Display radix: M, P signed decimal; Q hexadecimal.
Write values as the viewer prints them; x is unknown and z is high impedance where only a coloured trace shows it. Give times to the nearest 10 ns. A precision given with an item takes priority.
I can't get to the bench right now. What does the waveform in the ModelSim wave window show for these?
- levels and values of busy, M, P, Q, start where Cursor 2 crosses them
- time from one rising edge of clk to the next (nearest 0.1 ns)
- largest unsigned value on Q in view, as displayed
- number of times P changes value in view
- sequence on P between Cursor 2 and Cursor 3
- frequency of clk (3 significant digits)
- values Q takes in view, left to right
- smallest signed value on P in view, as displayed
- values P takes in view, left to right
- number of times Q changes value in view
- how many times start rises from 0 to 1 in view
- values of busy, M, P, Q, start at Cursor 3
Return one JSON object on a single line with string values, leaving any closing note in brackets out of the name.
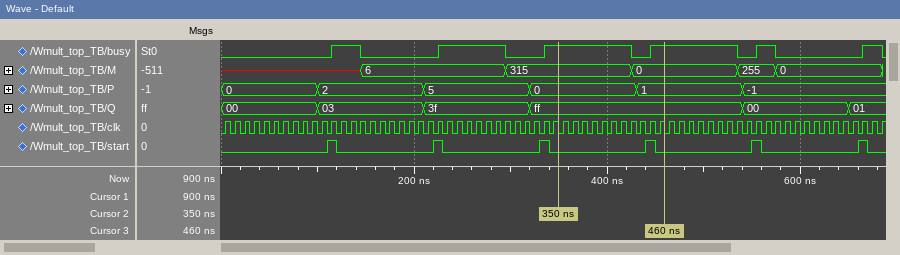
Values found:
{"levels and values of busy, M, P, Q, start where Cursor 2 crosses them": "busy=1, M=315, P=0, Q=ff, start=0", "time from one rising edge of clk to the next": "10 ns", "largest unsigned value on Q in view, as displayed": "ff", "number of times P changes value in view": "5", "sequence on P between Cursor 2 and Cursor 3": "0, 1", "frequency of clk": "100 MHz", "values Q takes in view, left to right": "00, 03, 3f, ff, 00, 01", "smallest signed value on P in view, as displayed": "-1", "values P takes in view, left to right": "0, 2, 5, 0, 1, -1", "number of times Q changes value in view": "5", "how many times start rises from 0 to 1 in view": "6", "values of busy, M, P, Q, start at Cursor 3": "busy=1, M=0, P=1, Q=ff, start=0"}
